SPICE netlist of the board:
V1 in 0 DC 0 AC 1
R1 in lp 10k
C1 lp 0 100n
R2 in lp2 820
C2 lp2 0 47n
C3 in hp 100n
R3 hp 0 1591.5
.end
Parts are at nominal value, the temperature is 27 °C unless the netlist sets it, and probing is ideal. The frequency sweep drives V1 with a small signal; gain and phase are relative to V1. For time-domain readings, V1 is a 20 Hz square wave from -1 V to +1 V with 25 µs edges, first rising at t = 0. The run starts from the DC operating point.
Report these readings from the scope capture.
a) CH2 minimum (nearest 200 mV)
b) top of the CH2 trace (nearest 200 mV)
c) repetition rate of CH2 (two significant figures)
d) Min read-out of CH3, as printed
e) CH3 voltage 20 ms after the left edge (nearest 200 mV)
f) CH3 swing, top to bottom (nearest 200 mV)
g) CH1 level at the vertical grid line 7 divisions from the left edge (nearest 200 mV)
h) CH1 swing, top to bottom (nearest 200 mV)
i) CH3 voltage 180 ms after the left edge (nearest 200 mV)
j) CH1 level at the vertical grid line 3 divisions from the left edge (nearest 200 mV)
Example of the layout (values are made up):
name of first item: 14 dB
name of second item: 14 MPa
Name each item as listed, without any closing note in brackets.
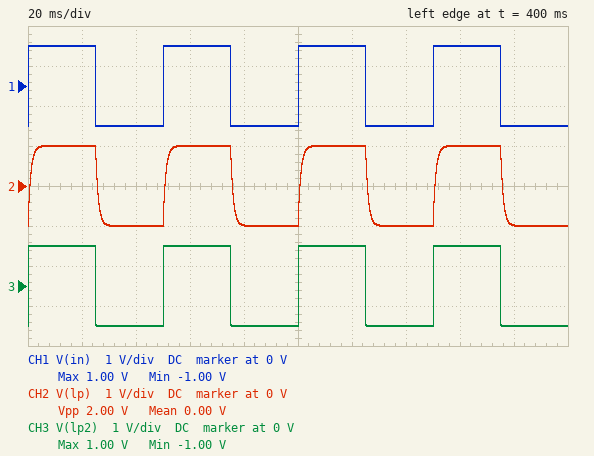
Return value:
CH2 minimum: -1.0 V
top of the CH2 trace: 1.0 V
repetition rate of CH2: 20 Hz
Min read-out of CH3, as printed: -1.00 V
CH3 voltage 20 ms after the left edge: 1.0 V
CH3 swing, top to bottom: 2.0 V
CH1 level at the vertical grid line 7 divisions from the left edge: -1.0 V
CH1 swing, top to bottom: 2.0 V
CH3 voltage 180 ms after the left edge: -1.0 V
CH1 level at the vertical grid line 3 divisions from the left edge: 1.0 V
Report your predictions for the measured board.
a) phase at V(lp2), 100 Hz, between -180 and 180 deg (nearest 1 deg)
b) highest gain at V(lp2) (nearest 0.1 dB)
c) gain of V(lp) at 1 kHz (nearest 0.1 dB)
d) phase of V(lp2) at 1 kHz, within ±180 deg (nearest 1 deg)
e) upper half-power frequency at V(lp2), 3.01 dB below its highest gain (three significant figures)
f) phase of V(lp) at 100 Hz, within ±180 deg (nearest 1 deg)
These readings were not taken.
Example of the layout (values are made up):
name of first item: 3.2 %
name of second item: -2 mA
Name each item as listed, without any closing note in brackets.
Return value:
phase at V(lp2), 100 Hz, between -180 and 180 deg: -1 deg
highest gain at V(lp2): 0 dB
gain of V(lp) at 1 kHz: -16.1 dB
phase of V(lp2) at 1 kHz, within ±180 deg: -14 deg
upper half-power frequency at V(lp2), 3.01 dB below its highest gain: 4.13 kHz
phase of V(lp) at 100 Hz, within ±180 deg: -32 deg
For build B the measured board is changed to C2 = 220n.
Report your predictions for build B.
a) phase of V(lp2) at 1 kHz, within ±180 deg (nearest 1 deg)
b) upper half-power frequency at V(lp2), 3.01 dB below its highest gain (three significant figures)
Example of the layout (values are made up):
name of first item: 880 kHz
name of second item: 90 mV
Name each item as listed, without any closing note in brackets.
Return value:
phase of V(lp2) at 1 kHz, within ±180 deg: -49 deg
upper half-power frequency at V(lp2), 3.01 dB below its highest gain: 882 Hz
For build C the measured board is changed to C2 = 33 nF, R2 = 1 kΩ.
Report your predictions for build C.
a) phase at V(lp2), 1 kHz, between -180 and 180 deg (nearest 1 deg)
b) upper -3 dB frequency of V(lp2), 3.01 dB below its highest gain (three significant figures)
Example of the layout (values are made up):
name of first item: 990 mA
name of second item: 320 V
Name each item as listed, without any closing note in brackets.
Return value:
phase at V(lp2), 1 kHz, between -180 and 180 deg: -12 deg
upper -3 dB frequency of V(lp2), 3.01 dB below its highest gain: 4.82 kHz
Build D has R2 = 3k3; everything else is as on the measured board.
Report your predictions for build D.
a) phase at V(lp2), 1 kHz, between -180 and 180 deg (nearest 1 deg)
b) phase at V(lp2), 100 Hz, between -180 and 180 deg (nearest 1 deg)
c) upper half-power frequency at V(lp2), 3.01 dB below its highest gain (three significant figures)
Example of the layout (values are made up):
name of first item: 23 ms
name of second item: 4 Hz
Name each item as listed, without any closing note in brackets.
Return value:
phase at V(lp2), 1 kHz, between -180 and 180 deg: -44 deg
phase at V(lp2), 100 Hz, between -180 and 180 deg: -6 deg
upper half-power frequency at V(lp2), 3.01 dB below its highest gain: 1.03 kHz
